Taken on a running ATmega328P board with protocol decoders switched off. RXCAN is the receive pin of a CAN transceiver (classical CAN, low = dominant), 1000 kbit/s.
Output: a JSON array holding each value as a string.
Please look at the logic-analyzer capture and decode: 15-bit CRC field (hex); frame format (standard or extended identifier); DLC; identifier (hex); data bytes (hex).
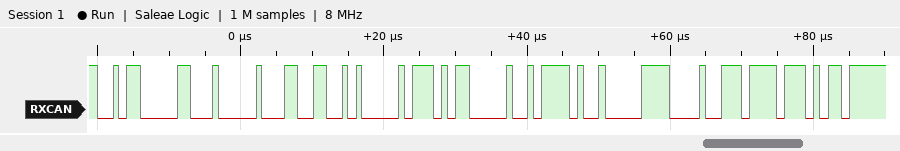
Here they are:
["0x6F75", "standard", "8", "0x2C1", "06 65 03 AC 05 E9 07 09"]
